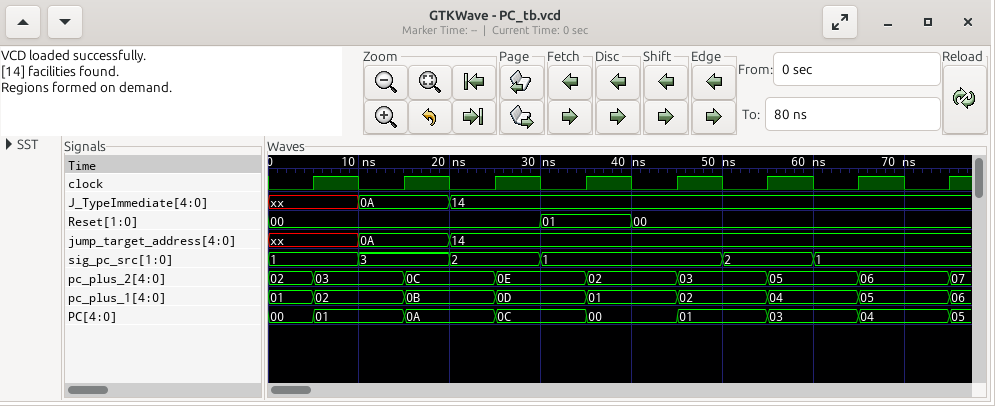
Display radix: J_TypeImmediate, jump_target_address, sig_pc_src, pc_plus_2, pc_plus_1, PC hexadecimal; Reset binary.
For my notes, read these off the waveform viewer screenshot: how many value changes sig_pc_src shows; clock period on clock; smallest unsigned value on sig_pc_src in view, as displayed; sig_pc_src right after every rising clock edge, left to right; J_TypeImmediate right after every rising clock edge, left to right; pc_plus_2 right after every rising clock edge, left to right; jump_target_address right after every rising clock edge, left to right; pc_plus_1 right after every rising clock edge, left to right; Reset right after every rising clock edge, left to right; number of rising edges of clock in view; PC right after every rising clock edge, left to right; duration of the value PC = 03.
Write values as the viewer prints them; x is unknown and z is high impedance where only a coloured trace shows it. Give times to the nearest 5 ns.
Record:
5
10 ns
1
1, 3, 2, 1, 1, 2, 1, 1
xx, 0A, 14, 14, 14, 14, 14, 14
03, 0C, 0E, 02, 03, 05, 06, 07
xx, 0A, 14, 14, 14, 14, 14, 14
02, 0B, 0D, 01, 02, 04, 05, 06
00, 00, 00, 01, 00, 00, 00, 00
8
01, 0A, 0C, 00, 01, 03, 04, 05
10 ns
